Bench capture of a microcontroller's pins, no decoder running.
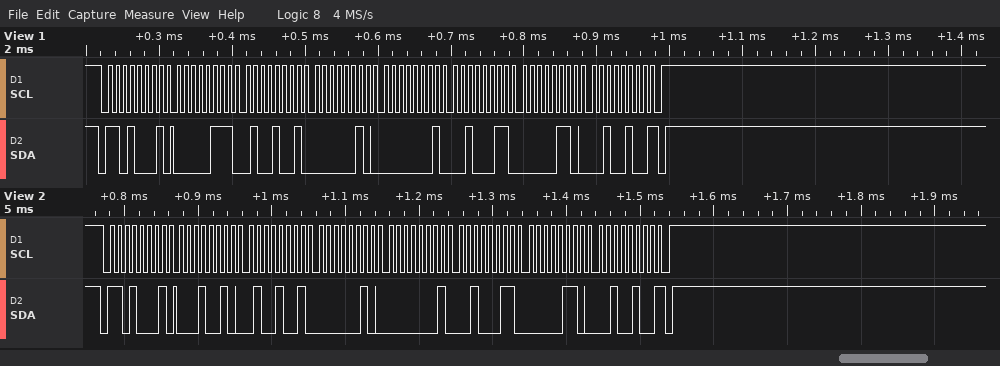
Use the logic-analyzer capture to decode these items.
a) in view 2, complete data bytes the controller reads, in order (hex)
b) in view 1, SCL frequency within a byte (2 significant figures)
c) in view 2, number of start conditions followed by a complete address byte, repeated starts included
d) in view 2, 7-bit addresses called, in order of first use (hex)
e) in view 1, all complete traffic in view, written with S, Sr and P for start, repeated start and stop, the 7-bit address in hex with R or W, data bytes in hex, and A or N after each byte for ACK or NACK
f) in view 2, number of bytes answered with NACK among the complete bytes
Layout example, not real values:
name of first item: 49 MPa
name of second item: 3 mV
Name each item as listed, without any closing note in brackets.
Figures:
in view 2, complete data bytes the controller reads, in order: 12 49 02 01 23 06 24
in view 1, SCL frequency within a byte: 100 kHz
in view 2, number of start conditions followed by a complete address byte, repeated starts included: 1
in view 2, 7-bit addresses called, in order of first use: 0x68
in view 1, all complete traffic in view, written with S, Sr and P for start, repeated start and stop, the 7-bit address in hex with R or W, data bytes in hex, and A or N after each byte for ACK or NACK: S 68R A 07 A 49 A 02 A 01 A 23 A 06 A 24 N P
in view 2, number of bytes answered with NACK among the complete bytes: 1
